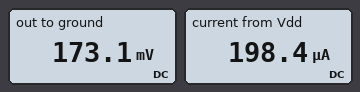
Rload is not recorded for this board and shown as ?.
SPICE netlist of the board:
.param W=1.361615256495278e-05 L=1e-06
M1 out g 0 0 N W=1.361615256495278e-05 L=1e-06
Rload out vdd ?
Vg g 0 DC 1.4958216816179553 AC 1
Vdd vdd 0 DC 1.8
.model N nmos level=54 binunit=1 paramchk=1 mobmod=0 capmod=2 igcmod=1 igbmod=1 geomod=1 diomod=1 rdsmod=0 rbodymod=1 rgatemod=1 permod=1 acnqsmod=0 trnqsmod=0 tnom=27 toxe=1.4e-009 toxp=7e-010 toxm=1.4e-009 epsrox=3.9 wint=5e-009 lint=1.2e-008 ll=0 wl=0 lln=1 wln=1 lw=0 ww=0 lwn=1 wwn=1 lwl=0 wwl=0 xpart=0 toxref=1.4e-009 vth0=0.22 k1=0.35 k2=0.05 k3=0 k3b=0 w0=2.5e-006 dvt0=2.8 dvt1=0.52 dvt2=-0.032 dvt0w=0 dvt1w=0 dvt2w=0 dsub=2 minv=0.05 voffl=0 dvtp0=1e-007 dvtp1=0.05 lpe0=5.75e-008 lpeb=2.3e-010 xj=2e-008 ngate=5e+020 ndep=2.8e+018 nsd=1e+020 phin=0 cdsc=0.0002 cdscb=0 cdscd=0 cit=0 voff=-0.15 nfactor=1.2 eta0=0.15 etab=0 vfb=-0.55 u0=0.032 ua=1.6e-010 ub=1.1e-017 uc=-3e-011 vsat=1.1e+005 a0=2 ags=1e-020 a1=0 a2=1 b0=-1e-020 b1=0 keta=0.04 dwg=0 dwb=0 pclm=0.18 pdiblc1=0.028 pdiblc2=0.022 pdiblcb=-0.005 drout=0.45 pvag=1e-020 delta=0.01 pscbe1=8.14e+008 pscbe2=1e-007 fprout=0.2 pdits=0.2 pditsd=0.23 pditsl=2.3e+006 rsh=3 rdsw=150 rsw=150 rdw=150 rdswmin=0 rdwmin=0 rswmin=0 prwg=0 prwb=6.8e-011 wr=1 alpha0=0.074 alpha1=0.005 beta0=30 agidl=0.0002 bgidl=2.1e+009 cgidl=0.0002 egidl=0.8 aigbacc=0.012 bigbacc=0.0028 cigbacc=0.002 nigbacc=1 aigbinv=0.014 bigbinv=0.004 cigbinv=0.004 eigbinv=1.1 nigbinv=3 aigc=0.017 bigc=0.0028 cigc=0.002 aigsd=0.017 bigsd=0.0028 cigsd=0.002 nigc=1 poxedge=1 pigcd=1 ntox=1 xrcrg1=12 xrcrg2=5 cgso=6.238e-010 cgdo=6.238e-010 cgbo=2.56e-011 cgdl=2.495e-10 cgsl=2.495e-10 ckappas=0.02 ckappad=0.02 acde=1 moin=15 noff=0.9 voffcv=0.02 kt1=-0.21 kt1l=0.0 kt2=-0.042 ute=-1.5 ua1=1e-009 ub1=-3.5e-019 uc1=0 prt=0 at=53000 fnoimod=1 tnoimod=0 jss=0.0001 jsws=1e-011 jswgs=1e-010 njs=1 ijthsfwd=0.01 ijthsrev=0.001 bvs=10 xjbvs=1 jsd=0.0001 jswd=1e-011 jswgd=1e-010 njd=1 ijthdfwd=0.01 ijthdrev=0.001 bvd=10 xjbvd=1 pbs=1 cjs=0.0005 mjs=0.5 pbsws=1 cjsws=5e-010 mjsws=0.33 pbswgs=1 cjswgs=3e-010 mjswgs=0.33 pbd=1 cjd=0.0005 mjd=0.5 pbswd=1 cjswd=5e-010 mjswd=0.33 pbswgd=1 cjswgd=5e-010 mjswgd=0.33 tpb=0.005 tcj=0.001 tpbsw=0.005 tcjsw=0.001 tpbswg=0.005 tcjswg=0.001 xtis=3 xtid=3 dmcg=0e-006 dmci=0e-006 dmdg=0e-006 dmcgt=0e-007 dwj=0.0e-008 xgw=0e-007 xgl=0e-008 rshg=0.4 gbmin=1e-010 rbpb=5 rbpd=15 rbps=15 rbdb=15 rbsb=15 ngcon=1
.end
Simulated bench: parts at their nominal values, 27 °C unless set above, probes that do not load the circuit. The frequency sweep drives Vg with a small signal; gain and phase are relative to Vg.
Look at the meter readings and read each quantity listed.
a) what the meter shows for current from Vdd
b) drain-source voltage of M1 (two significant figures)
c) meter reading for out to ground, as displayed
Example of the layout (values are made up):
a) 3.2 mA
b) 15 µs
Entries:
a) 198.4 µA
b) 170 mV
c) 173.1 mV
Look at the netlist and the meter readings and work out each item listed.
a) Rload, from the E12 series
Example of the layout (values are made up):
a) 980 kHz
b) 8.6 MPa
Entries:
a) 8.2 kΩ
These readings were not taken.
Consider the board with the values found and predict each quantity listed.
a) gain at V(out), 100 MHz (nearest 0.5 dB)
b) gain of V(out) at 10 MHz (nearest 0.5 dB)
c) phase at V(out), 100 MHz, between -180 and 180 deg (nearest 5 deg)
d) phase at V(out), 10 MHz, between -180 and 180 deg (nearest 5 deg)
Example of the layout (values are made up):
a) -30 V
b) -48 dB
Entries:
a) -16.5 dB
b) -28.0 dB
c) 65 deg
d) 20 deg
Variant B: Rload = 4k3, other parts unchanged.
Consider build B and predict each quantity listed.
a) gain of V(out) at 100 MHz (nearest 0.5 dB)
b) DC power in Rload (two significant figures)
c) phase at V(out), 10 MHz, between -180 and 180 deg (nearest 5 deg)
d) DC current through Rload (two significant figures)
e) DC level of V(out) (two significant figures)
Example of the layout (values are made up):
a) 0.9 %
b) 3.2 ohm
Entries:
a) -16.0 dB
b) 500 µW
c) 30 deg
d) 340 µA
e) 330 mV
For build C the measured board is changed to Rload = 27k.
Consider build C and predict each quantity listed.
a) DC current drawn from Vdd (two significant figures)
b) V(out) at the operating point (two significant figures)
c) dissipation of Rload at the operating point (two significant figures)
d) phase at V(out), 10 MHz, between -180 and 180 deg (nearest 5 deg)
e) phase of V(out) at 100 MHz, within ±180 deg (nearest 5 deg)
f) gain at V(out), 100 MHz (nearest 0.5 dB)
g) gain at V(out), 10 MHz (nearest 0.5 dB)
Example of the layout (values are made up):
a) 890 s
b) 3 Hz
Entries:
a) 65 µA
b) 55 mV
c) 110 µW
d) 25 deg
e) 70 deg
f) -17.0 dB
g) -30.5 dB
